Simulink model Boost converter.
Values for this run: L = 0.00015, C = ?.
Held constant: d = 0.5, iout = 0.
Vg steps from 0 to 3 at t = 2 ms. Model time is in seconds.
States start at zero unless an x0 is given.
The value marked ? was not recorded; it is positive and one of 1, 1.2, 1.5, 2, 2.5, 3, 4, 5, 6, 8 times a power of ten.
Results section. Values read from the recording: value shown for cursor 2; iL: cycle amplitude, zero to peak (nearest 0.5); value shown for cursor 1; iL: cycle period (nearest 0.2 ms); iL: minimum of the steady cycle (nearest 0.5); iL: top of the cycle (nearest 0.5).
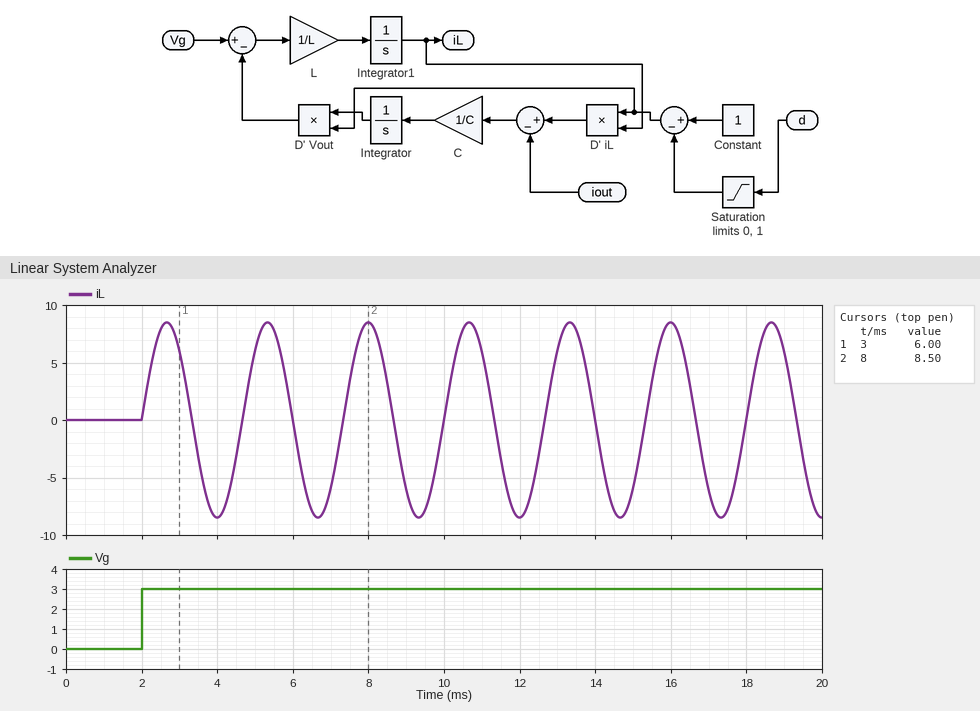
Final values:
8.50
8.5
6.00
2.6 ms
-8.5
8.5
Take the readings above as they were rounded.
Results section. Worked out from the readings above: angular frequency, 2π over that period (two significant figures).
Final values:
2.4 rad/ms
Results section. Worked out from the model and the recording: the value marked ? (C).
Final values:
0.0003
